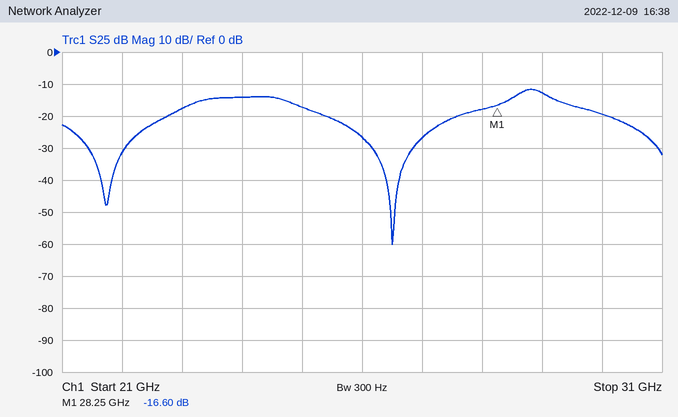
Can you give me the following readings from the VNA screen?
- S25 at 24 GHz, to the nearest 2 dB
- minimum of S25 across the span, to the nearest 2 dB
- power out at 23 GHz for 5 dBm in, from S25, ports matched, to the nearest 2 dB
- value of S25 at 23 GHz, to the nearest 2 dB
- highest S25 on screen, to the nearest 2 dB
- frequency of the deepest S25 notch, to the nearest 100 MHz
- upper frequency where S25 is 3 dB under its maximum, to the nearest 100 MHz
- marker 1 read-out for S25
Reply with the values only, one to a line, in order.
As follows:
-14 dB
-60 dB
-12 dBm
-18 dB
-12 dB
26.5 GHz
29.2 GHz
-16.60 dB
